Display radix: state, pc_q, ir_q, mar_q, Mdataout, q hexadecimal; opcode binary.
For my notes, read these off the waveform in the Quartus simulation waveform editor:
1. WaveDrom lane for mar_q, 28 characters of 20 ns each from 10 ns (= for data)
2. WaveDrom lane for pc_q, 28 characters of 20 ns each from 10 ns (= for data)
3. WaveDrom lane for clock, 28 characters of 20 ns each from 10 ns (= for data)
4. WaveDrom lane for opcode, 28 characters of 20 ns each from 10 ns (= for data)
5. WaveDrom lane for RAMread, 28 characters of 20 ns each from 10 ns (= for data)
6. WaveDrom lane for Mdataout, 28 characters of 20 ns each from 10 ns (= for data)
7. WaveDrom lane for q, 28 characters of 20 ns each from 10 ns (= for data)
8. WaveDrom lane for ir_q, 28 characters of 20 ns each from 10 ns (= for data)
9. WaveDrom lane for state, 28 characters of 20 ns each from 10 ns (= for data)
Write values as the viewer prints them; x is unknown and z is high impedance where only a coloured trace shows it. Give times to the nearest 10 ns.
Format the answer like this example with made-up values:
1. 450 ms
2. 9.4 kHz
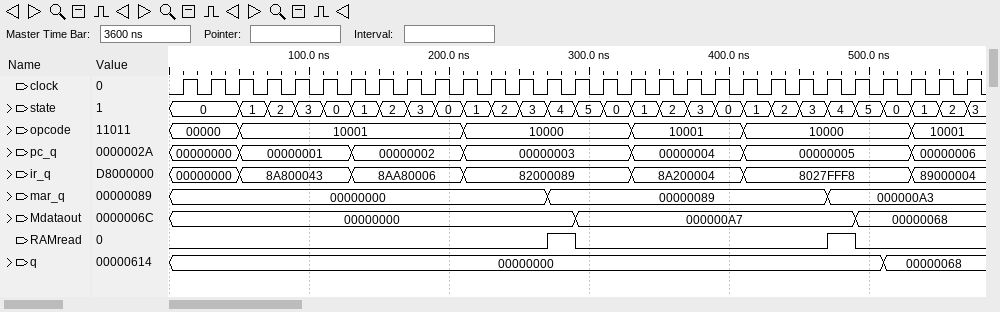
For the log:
1. {name: 'mar_q', wave: '=............=.........=....', data: '00000000 00000089 000000A3'}
2. {name: 'pc_q', wave: '=.=...=...=.....=...=.....=.', data: '00000000 00000001 00000002 00000003 00000004 00000005 00000006'}
3. {name: 'clock', wave: 'p...........................'}
4. {name: 'opcode', wave: '=.=.......=.....=...=.....=.', data: '00000 10001 10000 10001 10000 10001'}
5. {name: 'RAMread', wave: '0............10........10...'}
6. {name: 'Mdataout', wave: '=.............=.........=...', data: '00000000 000000A7 00000068'}
7. {name: 'q', wave: '=........................=..', data: '00000000 00000068'}
8. {name: 'ir_q', wave: '=.=...=...=.....=...=.....=.', data: '00000000 8A800043 8AA80006 82000089 8A200004 8027FFF8 89000004'}
9. {name: 'state', wave: '=.==========================', data: '0 1 2 3 0 1 2 3 0 1 2 3 4 5 0 1 2 3 0 1 2 3 4 5 0 1 2'}
